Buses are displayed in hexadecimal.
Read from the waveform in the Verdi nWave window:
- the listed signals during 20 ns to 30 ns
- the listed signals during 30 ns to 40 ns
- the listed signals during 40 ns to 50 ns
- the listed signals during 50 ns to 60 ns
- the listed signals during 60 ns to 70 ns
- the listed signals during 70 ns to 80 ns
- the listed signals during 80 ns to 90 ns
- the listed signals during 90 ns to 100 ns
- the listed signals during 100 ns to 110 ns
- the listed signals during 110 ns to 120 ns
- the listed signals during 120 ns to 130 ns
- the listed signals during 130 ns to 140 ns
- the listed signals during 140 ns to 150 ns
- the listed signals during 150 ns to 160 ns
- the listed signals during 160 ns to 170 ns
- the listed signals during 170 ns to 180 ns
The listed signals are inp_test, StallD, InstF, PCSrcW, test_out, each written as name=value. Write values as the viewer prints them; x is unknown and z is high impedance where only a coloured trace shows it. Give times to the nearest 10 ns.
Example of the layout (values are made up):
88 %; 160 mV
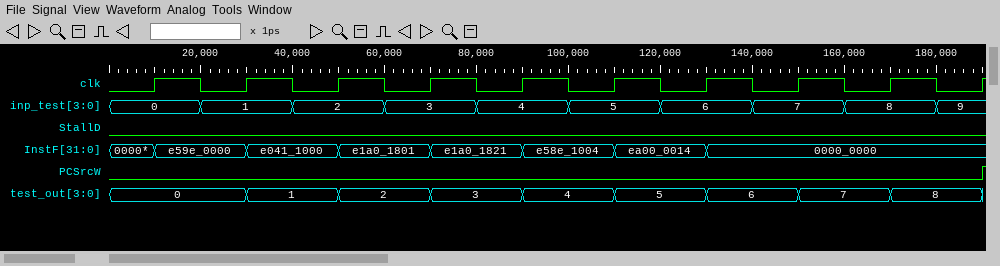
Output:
inp_test=1, StallD=0, InstF=e59e_0000, PCSrcW=0, test_out=0; inp_test=1, StallD=0, InstF=e041_1000, PCSrcW=0, test_out=1; inp_test=2, StallD=0, InstF=e041_1000, PCSrcW=0, test_out=1; inp_test=2, StallD=0, InstF=e1a0_1801, PCSrcW=0, test_out=2; inp_test=3, StallD=0, InstF=e1a0_1801, PCSrcW=0, test_out=2; inp_test=3, StallD=0, InstF=e1a0_1821, PCSrcW=0, test_out=3; inp_test=4, StallD=0, InstF=e1a0_1821, PCSrcW=0, test_out=3; inp_test=4, StallD=0, InstF=e58e_1004, PCSrcW=0, test_out=4; inp_test=5, StallD=0, InstF=e58e_1004, PCSrcW=0, test_out=4; inp_test=5, StallD=0, InstF=ea00_0014, PCSrcW=0, test_out=5; inp_test=6, StallD=0, InstF=ea00_0014, PCSrcW=0, test_out=5; inp_test=6, StallD=0, InstF=0000_0000, PCSrcW=0, test_out=6; inp_test=7, StallD=0, InstF=0000_0000, PCSrcW=0, test_out=6; inp_test=7, StallD=0, InstF=0000_0000, PCSrcW=0, test_out=7; inp_test=8, StallD=0, InstF=0000_0000, PCSrcW=0, test_out=7; inp_test=8, StallD=0, InstF=0000_0000, PCSrcW=0, test_out=8
